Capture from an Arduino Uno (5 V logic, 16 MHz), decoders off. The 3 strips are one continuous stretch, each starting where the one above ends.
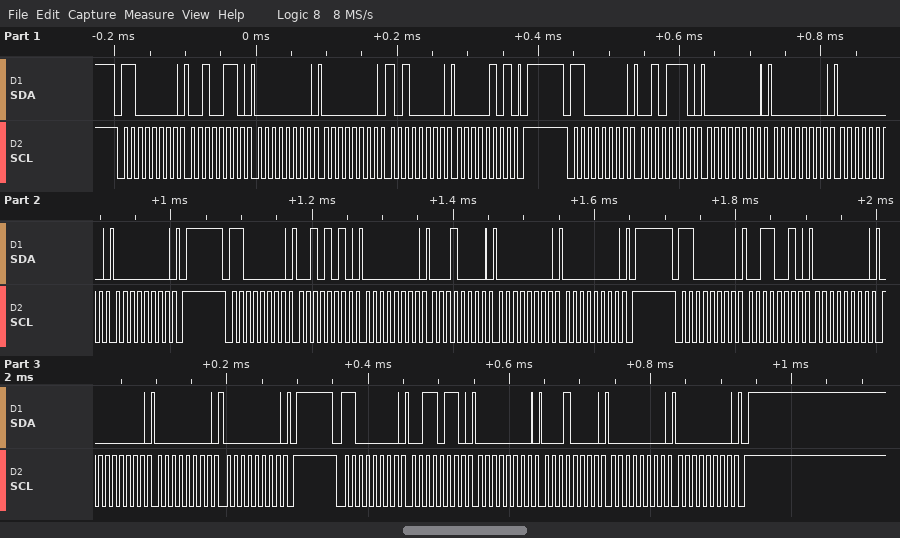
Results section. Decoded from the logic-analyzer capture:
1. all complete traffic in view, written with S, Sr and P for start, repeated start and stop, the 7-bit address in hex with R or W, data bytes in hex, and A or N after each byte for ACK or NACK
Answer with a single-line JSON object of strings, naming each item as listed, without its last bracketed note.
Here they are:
{"all complete traffic in view, written with S, Sr and P for start, repeated start and stop, the 7-bit address in hex with R or W, data bytes in hex, and A or N after each byte for ACK or NACK": "S 60W A 26 A 00 A 00 A A0 A 05 A P S 60W A 2E A 00 A 00 A 00 A 00 A P S 60W A 2A A 00 A 10 A 00 A 00 A P S 60W A 32 A 00 A 00 A 00 A 00 A P S 60W A 36 A 00 A 10 A 00 A 00 A P"}
